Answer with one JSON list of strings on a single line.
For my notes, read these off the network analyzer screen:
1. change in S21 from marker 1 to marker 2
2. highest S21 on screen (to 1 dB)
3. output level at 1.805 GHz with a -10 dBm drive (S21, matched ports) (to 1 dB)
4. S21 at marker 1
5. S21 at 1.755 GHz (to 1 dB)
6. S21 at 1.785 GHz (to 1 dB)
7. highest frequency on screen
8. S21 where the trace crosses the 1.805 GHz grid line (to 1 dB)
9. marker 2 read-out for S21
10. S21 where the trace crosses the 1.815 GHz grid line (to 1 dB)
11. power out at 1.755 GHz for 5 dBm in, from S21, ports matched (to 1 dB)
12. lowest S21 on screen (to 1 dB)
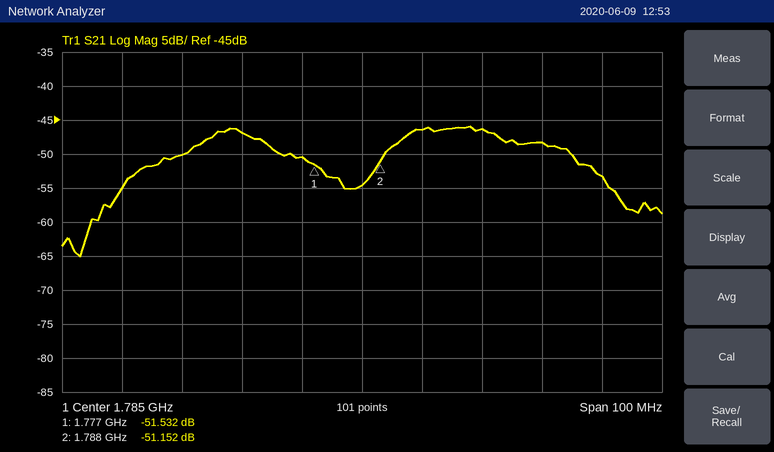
["0.380 dB", "-46 dB", "-56 dBm", "-51.532 dB", "-50 dB", "-55 dB", "1.835 GHz", "-46 dB", "-51.152 dB", "-48 dB", "-45 dBm", "-65 dB"]
